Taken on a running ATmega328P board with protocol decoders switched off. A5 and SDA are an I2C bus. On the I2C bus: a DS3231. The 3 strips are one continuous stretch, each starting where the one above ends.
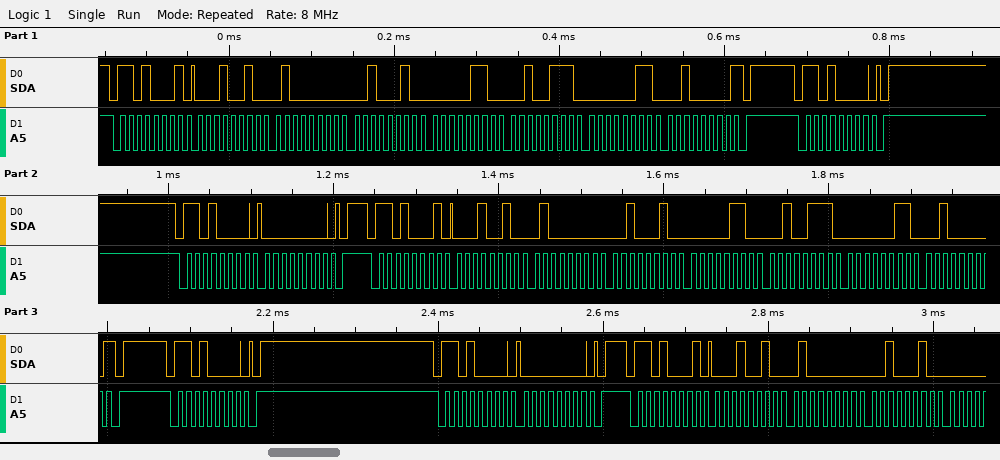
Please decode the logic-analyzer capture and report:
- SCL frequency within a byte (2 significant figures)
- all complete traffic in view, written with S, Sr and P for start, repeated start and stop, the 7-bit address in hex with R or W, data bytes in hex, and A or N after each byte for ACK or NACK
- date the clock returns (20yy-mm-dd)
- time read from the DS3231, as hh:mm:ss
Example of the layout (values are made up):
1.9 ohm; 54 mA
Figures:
100 kHz; S 68R A 12 A 40 A 22 A 06 A 27 A 03 A 20 N P S 68W A P S 68W A 00 A P S 68R A 12 A 40 A 22 A 06 A 27 A 03 A 20 N P S 68W A P S 68W A 00 A P S 68R A 12 A 40 A 22 A; 2020-03-27; 22:40:12
